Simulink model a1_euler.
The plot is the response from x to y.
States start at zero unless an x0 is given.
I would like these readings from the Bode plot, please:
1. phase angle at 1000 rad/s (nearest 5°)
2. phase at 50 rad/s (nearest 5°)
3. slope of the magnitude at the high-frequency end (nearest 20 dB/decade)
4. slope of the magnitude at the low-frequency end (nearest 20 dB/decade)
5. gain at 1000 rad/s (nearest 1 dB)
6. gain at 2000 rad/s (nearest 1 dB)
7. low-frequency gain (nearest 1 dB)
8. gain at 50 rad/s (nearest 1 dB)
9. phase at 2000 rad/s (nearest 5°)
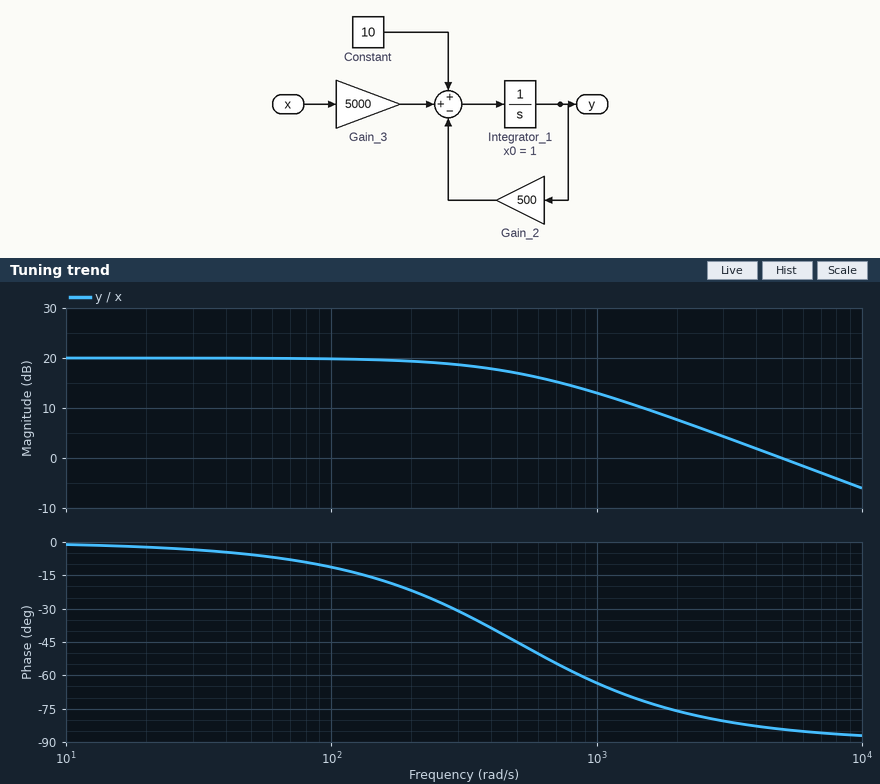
-65°
-5°
-20 dB/decade
0 dB/decade
13 dB
8 dB
20 dB
20 dB
-75°
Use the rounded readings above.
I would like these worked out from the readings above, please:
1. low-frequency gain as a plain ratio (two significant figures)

10
